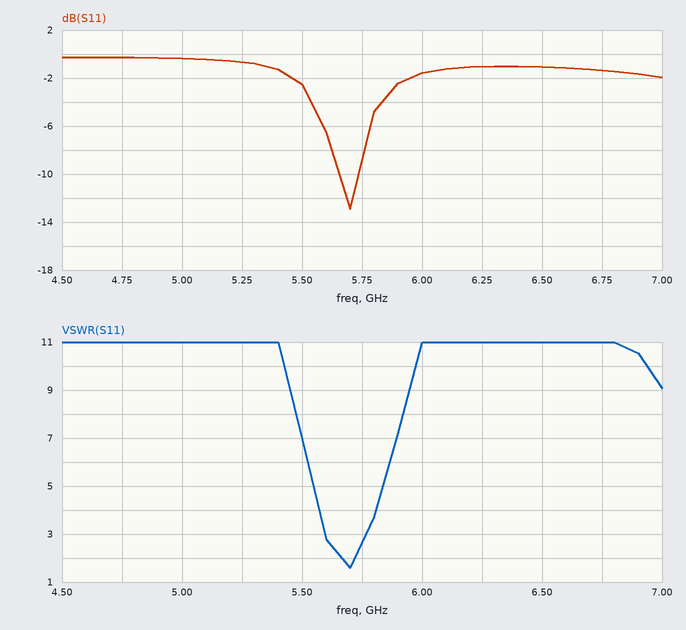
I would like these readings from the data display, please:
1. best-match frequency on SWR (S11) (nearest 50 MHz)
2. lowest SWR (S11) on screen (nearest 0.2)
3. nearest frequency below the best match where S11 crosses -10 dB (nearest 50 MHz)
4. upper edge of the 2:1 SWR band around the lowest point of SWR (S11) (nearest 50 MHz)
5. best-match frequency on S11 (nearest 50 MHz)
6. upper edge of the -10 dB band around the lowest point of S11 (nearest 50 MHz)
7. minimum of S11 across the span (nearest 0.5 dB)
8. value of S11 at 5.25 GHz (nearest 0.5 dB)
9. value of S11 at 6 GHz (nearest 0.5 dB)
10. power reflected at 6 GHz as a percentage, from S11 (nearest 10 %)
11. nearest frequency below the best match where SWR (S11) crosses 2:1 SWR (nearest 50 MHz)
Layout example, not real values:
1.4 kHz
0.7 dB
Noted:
5.70 GHz
1.6
5.65 GHz
5.70 GHz
5.70 GHz
5.75 GHz
-13.0 dB
-0.5 dB
-1.5 dB
70 %
5.65 GHz
